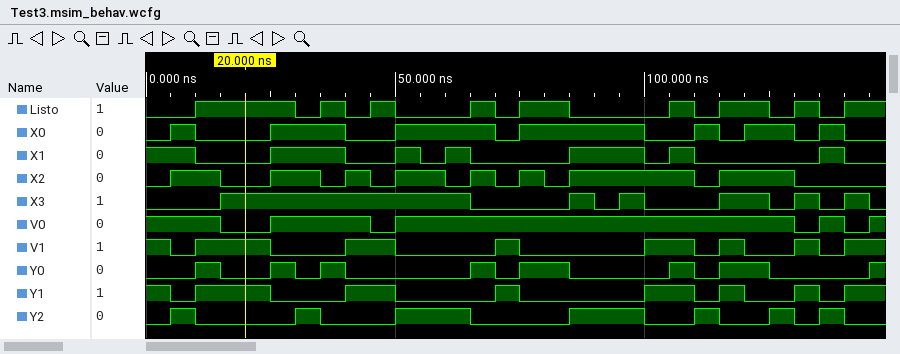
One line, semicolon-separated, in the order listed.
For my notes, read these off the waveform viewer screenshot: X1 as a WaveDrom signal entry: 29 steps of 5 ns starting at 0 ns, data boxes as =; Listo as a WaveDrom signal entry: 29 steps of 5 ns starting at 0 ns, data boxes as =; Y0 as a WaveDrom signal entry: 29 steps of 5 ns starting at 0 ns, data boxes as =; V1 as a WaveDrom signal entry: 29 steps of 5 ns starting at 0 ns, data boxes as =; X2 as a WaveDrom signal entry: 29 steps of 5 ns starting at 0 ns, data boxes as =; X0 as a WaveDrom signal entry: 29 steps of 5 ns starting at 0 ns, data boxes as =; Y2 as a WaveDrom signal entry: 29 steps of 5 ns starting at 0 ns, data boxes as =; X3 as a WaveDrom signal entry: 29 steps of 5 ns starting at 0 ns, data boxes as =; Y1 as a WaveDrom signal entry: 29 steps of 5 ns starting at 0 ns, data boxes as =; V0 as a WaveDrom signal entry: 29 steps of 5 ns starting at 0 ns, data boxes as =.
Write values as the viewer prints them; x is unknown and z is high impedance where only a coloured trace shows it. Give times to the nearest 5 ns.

{name: 'X1', wave: '1.0..1..0.1010...1..010....10'}; {name: 'Listo', wave: '0.1...01010..101.0...101.0101'}; {name: 'Y0', wave: '0.10.1010....101.0...101.0...'}; {name: 'V1', wave: '101..0..1.0...10....1.010.101'}; {name: 'X2', wave: '01.0.1.0101.010101....01..0..'}; {name: 'X0', wave: '010..1..0.1...01....0.101.010'}; {name: 'Y2', wave: '010...10..1..0...1..0.10.1010'}; {name: 'X3', wave: '0..1.........0...1010..1.0101'}; {name: 'Y1', wave: '101..0..1.0...10....1.010.101'}; {name: 'V0', wave: '1..0.1...01...............010'}
